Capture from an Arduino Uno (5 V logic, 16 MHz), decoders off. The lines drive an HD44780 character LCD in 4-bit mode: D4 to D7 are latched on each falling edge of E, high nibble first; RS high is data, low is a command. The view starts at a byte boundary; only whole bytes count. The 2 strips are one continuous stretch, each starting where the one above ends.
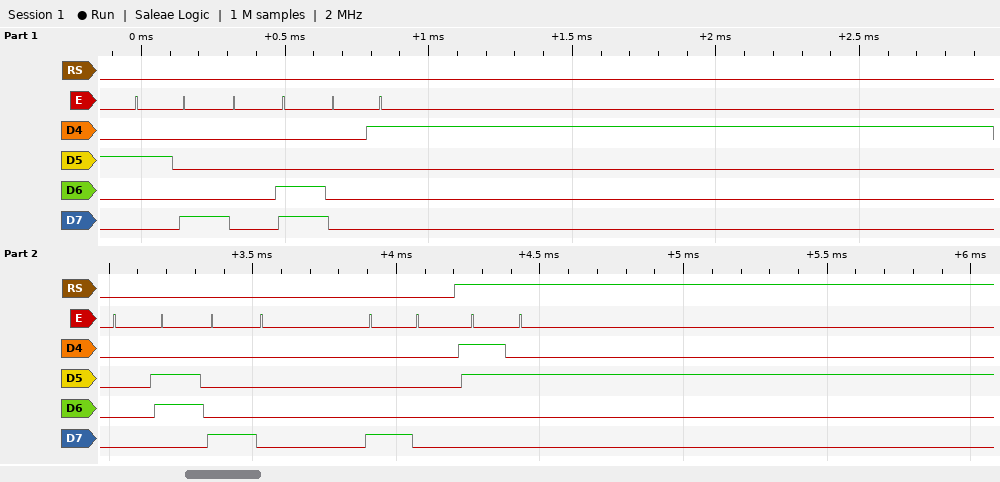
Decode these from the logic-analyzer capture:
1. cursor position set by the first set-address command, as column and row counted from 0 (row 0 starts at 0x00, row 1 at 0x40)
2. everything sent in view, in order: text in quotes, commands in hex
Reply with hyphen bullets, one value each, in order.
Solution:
- column 0, row 0
- 0x28 0x0C 0x01 0x06 0x80 0x80 "2"
